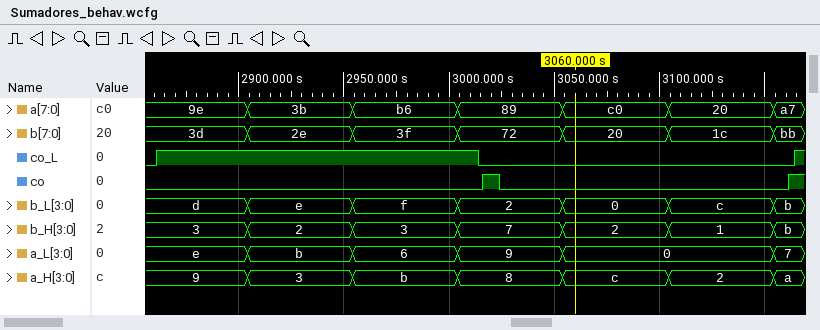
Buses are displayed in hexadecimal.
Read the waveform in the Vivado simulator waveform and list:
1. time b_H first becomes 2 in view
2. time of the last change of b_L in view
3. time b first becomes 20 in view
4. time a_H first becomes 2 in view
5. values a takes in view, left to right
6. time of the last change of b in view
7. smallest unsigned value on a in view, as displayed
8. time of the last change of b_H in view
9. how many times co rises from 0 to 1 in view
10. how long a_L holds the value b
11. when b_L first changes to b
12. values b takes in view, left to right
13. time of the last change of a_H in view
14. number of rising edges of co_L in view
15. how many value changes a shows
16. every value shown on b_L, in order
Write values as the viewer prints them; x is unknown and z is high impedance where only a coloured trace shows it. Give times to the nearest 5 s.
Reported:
2905 s
3155 s
3055 s
3105 s
9e, 3b, b6, 89, c0, 20, a7
3155 s
20
3155 s
2
50 s
3155 s
3d, 2e, 3f, 72, 20, 1c, bb
3155 s
2
6
d, e, f, 2, 0, c, b
